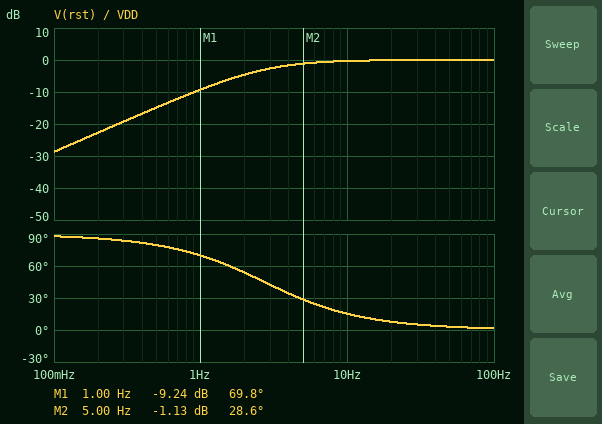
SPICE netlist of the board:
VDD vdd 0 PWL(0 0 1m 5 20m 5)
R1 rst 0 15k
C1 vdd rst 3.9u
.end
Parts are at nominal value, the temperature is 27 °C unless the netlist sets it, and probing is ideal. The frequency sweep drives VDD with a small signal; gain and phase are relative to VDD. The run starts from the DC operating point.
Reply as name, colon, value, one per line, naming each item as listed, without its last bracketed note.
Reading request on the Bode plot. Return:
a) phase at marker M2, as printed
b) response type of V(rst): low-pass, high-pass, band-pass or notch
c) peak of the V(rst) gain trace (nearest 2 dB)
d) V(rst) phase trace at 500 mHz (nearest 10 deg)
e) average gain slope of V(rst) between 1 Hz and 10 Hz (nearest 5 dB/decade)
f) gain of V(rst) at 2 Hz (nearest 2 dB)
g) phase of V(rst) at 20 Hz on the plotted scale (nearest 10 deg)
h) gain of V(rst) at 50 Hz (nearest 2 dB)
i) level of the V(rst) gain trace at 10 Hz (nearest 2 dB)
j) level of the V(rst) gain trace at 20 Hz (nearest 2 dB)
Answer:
phase at marker M2, as printed: 28.6 deg
response type of V(rst): low-pass, high-pass, band-pass or notch: high-pass
peak of the V(rst) gain trace: 0 dB
V(rst) phase trace at 500 mHz: 80 deg
average gain slope of V(rst) between 1 Hz and 10 Hz: 10 dB/decade
gain of V(rst) at 2 Hz: -4 dB
phase of V(rst) at 20 Hz on the plotted scale: 10 deg
gain of V(rst) at 50 Hz: 0 dB
level of the V(rst) gain trace at 10 Hz: 0 dB
level of the V(rst) gain trace at 20 Hz: 0 dB
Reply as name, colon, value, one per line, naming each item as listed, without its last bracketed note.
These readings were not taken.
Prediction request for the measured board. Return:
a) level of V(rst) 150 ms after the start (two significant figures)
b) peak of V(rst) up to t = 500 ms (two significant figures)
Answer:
level of V(rst) 150 ms after the start: 390 mV
peak of V(rst) up to t = 500 ms: 5.0 V
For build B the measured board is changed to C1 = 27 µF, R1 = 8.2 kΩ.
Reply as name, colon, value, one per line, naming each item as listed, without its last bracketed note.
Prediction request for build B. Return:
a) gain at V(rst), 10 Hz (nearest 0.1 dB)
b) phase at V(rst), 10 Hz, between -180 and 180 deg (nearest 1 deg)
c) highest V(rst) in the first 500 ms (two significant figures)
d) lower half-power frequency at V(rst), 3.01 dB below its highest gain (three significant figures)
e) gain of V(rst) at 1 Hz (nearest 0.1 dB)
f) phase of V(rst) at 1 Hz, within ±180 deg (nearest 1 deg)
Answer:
gain at V(rst), 10 Hz: 0 dB
phase at V(rst), 10 Hz, between -180 and 180 deg: 4 deg
highest V(rst) in the first 500 ms: 5.0 V
lower half-power frequency at V(rst), 3.01 dB below its highest gain: 719 mHz
gain of V(rst) at 1 Hz: -1.8 dB
phase of V(rst) at 1 Hz, within ±180 deg: 36 deg
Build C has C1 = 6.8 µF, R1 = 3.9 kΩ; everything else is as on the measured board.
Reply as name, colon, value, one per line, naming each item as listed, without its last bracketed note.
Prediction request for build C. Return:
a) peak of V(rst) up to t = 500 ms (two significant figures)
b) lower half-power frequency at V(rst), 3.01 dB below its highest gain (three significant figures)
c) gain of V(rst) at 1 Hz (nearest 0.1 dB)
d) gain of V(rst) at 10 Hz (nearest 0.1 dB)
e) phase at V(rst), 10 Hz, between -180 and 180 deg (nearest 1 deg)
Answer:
peak of V(rst) up to t = 500 ms: 4.9 V
lower half-power frequency at V(rst), 3.01 dB below its highest gain: 6.00 Hz
gain of V(rst) at 1 Hz: -15.7 dB
gain of V(rst) at 10 Hz: -1.3 dB
phase at V(rst), 10 Hz, between -180 and 180 deg: 31 deg
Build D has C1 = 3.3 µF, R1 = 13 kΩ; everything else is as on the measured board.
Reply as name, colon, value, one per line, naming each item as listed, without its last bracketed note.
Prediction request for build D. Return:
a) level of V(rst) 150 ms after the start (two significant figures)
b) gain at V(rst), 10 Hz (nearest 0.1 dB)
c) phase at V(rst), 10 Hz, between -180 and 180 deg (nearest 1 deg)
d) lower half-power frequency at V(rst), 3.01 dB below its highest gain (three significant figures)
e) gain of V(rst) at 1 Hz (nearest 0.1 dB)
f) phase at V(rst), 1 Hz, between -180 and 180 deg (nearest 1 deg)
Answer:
level of V(rst) 150 ms after the start: 150 mV
gain at V(rst), 10 Hz: -0.6 dB
phase at V(rst), 10 Hz, between -180 and 180 deg: 20 deg
lower half-power frequency at V(rst), 3.01 dB below its highest gain: 3.71 Hz
gain of V(rst) at 1 Hz: -11.7 dB
phase at V(rst), 1 Hz, between -180 and 180 deg: 75 deg
